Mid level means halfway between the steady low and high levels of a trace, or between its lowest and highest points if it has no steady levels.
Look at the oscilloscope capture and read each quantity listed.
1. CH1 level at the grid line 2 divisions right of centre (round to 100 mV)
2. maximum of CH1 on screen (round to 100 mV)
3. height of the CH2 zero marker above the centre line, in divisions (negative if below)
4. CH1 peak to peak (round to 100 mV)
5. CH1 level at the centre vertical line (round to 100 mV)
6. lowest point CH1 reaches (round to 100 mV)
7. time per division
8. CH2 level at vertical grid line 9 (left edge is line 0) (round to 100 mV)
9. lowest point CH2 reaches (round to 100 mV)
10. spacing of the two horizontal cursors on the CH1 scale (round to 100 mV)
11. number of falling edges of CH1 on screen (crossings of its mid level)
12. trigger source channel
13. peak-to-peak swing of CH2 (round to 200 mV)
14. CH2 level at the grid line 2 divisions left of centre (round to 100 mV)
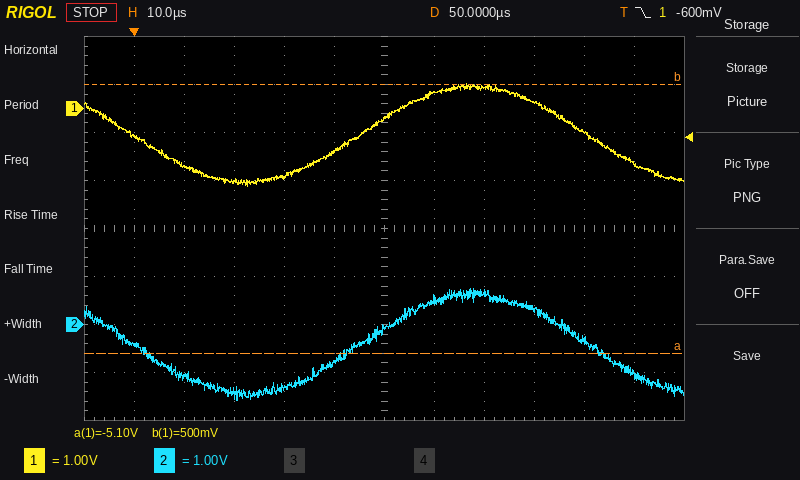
400 mV
500 mV
-2.0 div
2.1 V
-200 mV
-1.6 V
10 µs
300 mV
-1.6 V
5.6 V
2
CH1
2.4 V
-1.3 V
